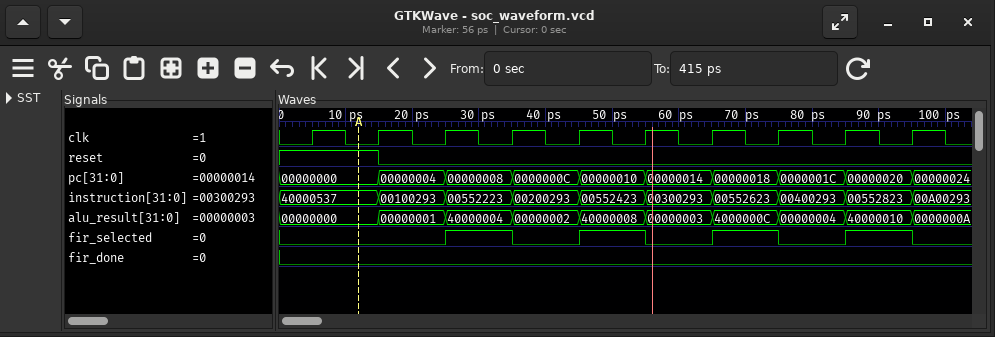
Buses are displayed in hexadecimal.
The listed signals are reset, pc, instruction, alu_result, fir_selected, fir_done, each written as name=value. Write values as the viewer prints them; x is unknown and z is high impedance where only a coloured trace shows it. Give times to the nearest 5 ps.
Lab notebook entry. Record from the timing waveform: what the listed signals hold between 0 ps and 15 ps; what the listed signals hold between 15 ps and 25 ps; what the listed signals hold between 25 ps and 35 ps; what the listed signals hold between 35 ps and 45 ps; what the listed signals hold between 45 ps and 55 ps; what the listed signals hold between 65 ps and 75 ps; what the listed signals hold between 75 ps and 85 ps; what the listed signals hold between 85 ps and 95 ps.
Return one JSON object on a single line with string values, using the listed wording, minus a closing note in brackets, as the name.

{"what the listed signals hold between 0 ps and 15 ps": "reset=1, pc=00000000, instruction=40000537, alu_result=00000000, fir_selected=0, fir_done=0", "what the listed signals hold between 15 ps and 25 ps": "reset=0, pc=00000004, instruction=00100293, alu_result=00000001, fir_selected=0, fir_done=0", "what the listed signals hold between 25 ps and 35 ps": "reset=0, pc=00000008, instruction=00552223, alu_result=40000004, fir_selected=1, fir_done=0", "what the listed signals hold between 35 ps and 45 ps": "reset=0, pc=0000000C, instruction=00200293, alu_result=00000002, fir_selected=0, fir_done=0", "what the listed signals hold between 45 ps and 55 ps": "reset=0, pc=00000010, instruction=00552423, alu_result=40000008, fir_selected=1, fir_done=0", "what the listed signals hold between 65 ps and 75 ps": "reset=0, pc=00000018, instruction=00552623, alu_result=4000000C, fir_selected=1, fir_done=0", "what the listed signals hold between 75 ps and 85 ps": "reset=0, pc=0000001C, instruction=00400293, alu_result=00000004, fir_selected=0, fir_done=0", "what the listed signals hold between 85 ps and 95 ps": "reset=0, pc=00000020, instruction=00552823, alu_result=40000010, fir_selected=1, fir_done=0"}
